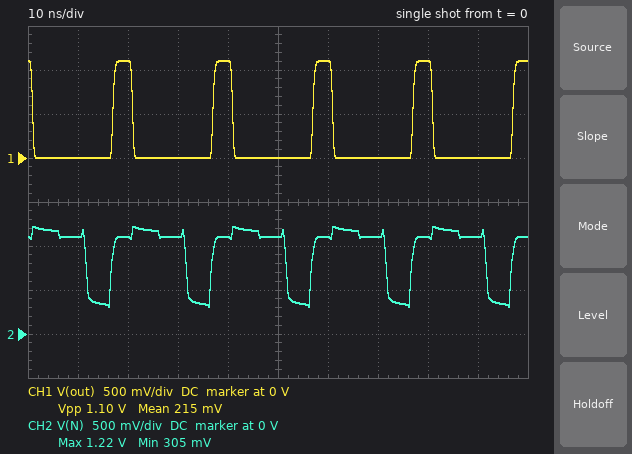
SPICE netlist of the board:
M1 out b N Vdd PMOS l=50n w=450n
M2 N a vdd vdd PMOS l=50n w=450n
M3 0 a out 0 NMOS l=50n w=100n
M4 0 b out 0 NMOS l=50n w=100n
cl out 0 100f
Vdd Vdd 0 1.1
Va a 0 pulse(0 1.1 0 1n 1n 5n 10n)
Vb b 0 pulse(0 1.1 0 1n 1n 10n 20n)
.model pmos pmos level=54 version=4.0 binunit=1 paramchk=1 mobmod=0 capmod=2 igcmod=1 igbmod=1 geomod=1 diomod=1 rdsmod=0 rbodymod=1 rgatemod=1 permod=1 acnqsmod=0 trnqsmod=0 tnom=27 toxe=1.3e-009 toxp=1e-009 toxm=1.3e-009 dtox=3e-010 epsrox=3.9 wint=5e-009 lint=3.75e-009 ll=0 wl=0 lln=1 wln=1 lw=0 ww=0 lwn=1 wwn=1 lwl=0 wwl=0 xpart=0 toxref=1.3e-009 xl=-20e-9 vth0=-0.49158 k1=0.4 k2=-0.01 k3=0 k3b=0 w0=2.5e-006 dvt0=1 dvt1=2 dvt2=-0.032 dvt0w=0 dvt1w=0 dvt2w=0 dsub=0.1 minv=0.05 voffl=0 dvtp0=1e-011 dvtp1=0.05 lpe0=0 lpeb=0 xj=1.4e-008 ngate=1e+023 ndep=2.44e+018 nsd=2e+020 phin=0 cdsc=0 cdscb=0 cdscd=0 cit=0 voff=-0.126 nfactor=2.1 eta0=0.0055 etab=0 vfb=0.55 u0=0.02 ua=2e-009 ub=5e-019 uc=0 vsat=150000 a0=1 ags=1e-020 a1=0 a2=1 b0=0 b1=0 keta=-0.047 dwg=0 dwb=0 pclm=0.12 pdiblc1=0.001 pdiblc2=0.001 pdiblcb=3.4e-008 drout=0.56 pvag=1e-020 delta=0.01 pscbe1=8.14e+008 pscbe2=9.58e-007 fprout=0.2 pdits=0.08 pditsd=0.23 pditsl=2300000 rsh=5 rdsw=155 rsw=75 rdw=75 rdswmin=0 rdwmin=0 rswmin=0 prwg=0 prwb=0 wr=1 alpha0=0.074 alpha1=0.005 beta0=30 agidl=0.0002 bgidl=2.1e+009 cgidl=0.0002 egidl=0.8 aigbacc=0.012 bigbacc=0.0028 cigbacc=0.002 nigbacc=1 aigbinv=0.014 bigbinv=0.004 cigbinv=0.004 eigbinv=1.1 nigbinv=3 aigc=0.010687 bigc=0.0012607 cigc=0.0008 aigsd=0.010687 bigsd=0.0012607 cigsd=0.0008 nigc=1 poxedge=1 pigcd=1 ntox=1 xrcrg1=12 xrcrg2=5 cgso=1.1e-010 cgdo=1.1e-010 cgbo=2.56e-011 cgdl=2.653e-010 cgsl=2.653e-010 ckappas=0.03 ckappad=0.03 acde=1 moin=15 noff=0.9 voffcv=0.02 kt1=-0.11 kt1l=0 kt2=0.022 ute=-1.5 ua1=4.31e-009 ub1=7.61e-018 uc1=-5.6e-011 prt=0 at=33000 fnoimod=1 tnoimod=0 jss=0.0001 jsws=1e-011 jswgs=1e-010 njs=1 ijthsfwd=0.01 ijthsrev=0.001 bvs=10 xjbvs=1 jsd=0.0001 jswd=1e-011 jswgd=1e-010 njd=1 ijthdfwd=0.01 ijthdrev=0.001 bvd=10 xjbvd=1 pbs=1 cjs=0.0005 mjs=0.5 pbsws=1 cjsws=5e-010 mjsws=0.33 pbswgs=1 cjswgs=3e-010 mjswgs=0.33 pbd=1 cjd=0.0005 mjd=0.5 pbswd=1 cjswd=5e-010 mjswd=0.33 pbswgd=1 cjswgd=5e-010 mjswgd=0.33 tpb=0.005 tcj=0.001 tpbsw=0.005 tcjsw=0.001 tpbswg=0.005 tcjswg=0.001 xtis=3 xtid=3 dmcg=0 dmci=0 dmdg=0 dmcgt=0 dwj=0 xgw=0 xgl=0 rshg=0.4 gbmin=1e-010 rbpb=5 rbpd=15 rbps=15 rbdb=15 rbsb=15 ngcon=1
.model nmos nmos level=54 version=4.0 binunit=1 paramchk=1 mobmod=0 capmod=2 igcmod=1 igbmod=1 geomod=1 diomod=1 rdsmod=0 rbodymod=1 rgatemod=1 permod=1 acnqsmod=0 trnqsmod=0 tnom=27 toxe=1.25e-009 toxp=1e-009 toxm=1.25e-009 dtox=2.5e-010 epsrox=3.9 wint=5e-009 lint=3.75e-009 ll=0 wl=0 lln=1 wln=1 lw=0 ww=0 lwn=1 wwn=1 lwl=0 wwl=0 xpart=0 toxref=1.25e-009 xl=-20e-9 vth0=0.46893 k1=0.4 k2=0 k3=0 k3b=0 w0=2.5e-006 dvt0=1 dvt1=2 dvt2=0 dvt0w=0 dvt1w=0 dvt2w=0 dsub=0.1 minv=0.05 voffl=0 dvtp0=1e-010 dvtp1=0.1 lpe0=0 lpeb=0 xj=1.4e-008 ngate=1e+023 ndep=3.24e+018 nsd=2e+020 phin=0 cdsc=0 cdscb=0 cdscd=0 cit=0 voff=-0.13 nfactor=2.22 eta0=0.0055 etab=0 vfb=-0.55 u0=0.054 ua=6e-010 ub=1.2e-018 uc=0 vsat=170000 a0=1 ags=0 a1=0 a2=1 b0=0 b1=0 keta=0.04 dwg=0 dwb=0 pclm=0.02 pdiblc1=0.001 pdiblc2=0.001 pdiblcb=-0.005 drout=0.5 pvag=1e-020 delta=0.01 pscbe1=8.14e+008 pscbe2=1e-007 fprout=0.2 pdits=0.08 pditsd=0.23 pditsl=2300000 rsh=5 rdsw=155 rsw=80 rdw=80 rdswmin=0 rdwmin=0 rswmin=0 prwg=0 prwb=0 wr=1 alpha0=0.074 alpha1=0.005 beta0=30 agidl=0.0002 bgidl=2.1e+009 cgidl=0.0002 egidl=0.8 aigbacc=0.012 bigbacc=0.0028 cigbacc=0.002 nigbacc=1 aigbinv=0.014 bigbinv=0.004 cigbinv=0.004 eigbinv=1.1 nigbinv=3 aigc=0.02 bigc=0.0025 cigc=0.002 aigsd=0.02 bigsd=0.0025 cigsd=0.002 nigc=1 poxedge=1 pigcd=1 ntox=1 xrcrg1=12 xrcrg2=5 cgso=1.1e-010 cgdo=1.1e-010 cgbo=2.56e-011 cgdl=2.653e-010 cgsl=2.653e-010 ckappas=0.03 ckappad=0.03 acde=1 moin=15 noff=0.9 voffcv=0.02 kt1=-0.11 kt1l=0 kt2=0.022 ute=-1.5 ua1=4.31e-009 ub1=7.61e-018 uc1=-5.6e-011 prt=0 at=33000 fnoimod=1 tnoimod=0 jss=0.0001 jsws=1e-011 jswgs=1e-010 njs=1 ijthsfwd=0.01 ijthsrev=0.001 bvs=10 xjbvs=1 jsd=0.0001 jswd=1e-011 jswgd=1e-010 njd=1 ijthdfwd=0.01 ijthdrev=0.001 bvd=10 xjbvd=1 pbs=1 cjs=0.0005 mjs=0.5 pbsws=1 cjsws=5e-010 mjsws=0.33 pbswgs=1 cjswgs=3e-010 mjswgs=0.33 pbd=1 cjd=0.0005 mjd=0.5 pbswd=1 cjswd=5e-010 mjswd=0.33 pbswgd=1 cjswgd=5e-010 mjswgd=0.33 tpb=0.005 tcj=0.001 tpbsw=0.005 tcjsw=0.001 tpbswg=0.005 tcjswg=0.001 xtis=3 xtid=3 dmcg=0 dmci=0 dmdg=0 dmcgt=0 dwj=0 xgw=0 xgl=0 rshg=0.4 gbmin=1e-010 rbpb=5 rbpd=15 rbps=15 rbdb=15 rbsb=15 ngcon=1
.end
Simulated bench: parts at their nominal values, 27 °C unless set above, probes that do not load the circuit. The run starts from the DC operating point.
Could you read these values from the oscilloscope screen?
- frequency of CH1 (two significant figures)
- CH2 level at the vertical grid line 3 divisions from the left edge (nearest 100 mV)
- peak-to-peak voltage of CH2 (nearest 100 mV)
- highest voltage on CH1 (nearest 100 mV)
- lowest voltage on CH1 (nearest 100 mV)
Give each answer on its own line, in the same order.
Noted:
50 MHz
1.1 V
900 mV
1.1 V
0 V
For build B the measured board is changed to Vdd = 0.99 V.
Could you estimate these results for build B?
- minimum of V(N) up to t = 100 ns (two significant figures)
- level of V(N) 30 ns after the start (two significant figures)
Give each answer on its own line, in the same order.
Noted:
270 mV
990 mV
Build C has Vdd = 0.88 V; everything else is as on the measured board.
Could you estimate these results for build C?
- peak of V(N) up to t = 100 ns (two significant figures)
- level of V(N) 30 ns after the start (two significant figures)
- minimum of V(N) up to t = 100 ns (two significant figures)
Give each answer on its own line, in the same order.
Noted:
1.1 V
880 mV
240 mV
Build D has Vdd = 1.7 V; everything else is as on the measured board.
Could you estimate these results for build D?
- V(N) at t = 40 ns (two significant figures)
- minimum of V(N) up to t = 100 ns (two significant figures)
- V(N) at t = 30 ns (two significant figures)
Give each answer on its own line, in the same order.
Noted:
1.7 V
790 mV
1.6 V
